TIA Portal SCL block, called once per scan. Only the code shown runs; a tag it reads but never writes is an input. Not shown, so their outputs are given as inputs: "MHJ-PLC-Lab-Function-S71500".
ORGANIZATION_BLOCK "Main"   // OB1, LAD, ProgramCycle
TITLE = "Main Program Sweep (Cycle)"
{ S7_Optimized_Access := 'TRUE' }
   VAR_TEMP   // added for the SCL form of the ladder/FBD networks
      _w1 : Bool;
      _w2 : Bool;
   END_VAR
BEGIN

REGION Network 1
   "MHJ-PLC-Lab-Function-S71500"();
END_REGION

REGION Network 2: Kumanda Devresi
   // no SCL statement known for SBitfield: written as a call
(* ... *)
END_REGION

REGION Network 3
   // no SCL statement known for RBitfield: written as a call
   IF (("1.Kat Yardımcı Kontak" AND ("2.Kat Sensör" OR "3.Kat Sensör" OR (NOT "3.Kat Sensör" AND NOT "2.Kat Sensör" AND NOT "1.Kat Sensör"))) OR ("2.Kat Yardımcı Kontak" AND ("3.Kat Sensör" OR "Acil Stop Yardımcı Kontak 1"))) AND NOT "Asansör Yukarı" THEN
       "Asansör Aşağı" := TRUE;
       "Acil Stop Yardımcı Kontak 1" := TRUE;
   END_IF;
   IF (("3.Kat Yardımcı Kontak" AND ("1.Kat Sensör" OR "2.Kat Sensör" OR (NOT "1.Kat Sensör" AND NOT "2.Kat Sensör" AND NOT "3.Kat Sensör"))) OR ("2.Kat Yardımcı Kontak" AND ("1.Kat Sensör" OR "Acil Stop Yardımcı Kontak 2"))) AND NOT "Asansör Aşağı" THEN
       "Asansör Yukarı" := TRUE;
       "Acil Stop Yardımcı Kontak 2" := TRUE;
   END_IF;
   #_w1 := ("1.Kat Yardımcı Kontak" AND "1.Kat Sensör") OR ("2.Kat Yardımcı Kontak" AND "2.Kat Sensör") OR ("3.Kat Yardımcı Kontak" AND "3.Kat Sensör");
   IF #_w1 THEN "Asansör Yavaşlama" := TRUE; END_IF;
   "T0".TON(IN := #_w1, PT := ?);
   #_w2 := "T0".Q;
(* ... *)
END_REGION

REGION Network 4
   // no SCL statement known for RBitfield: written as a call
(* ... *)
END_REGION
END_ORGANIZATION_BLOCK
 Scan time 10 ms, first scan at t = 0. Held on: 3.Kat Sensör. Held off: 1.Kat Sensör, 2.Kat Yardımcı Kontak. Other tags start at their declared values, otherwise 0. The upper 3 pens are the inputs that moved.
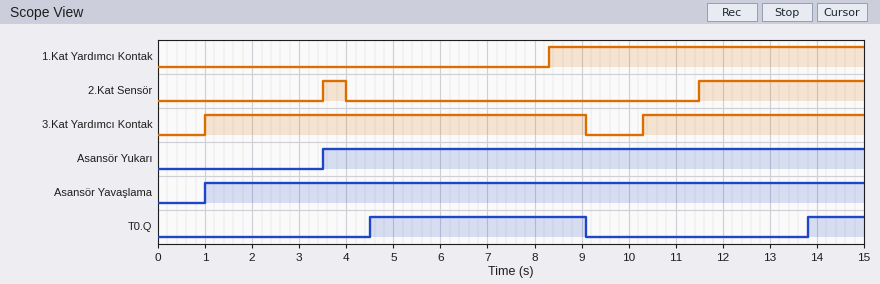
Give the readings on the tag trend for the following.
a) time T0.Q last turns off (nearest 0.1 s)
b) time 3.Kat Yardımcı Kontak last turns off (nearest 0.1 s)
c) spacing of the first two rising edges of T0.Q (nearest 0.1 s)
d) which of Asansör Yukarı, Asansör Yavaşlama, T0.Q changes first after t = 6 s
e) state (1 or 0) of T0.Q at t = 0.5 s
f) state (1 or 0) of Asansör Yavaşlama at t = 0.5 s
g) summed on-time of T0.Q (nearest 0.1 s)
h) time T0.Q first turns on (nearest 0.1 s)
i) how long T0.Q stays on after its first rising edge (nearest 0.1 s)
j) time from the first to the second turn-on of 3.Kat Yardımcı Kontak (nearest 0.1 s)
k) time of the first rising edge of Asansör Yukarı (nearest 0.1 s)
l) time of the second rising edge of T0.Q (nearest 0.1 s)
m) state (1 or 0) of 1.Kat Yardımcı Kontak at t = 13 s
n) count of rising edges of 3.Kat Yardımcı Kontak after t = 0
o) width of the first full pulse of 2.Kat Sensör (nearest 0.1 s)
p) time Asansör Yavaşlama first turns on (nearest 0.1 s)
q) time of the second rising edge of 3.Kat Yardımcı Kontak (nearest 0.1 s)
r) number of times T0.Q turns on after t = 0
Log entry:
9.1 s
9.1 s
9.3 s
T0.Q
0
0
5.8 s
4.5 s
4.6 s
9.3 s
3.5 s
13.8 s
1
2
0.5 s
1.0 s
10.3 s
2
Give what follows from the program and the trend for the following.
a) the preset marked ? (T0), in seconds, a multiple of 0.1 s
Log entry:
3.5 s
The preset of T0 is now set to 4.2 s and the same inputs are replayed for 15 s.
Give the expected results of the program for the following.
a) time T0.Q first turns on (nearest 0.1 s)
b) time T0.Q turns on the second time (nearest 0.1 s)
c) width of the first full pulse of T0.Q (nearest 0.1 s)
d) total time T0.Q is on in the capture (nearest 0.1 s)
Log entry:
5.2 s
14.5 s
3.9 s
4.4 s
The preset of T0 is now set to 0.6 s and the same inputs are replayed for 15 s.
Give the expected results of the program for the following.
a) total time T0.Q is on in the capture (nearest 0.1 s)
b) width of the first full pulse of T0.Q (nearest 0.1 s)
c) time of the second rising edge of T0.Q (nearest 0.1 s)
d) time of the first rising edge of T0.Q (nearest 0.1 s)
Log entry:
11.6 s
7.5 s
10.9 s
1.6 s
